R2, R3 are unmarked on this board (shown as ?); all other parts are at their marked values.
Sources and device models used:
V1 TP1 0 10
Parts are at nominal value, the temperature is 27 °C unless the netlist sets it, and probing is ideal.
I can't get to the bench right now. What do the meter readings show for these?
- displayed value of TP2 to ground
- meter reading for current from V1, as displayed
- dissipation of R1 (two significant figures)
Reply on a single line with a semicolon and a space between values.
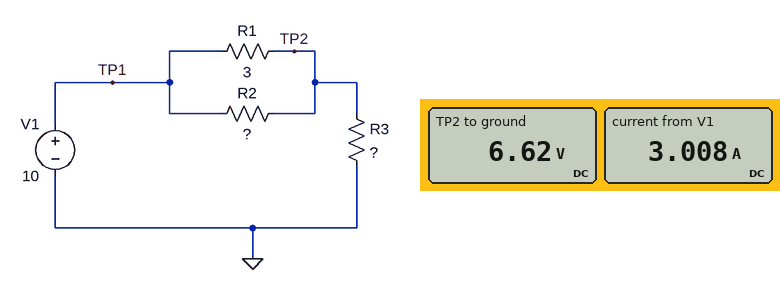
6.62 V; 3.008 A; 3.8 W
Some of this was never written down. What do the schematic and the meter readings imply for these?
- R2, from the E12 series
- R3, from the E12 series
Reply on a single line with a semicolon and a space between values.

1.8 Ω; 2.2 Ω
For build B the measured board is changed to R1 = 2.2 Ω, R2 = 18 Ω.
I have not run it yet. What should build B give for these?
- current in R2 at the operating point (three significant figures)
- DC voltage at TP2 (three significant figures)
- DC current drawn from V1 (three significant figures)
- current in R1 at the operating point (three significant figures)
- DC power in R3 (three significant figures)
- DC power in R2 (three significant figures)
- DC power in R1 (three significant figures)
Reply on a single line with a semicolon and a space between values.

262 mA; 5.29 V; 2.40 A; 2.14 A; 12.7 W; 1.23 W; 10.1 W
